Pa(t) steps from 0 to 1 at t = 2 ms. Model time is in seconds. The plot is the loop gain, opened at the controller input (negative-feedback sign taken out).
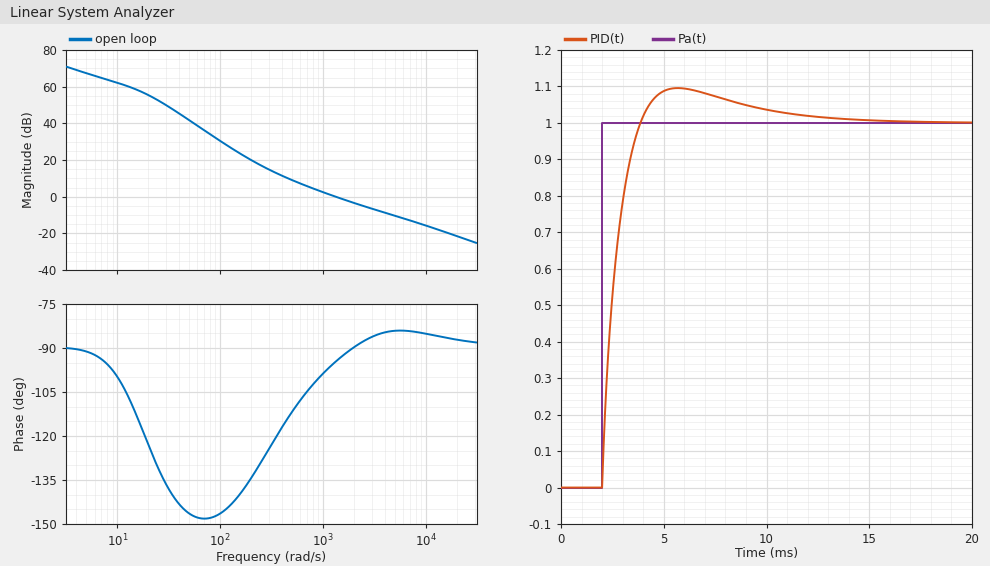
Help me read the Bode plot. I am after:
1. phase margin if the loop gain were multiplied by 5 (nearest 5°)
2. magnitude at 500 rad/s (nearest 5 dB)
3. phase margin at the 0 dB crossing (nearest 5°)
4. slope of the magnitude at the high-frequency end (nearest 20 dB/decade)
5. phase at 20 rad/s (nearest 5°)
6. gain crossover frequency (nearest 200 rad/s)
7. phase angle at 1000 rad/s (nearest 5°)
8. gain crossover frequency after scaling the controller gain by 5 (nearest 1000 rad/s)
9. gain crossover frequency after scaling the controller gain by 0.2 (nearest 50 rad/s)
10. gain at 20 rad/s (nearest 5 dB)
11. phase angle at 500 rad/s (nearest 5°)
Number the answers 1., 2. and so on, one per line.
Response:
1. 95°
2. 10 dB
3. 85°
4. -20 dB/decade
5. -125°
6. 1400 rad/s
7. -100°
8. 8000 rad/s
9. 300 rad/s
10. 55 dB
11. -110°
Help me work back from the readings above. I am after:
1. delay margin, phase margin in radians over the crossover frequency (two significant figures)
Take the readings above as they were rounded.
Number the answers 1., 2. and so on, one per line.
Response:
1. 0.0011 s
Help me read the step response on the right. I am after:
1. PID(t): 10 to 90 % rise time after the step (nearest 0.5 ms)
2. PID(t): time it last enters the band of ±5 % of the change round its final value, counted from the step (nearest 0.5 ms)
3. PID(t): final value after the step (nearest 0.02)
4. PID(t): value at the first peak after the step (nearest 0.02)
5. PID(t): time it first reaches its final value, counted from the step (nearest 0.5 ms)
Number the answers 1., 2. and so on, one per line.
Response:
1. 1.5 ms
2. 7.0 ms
3. 1.00
4. 1.10
5. 2.0 ms
